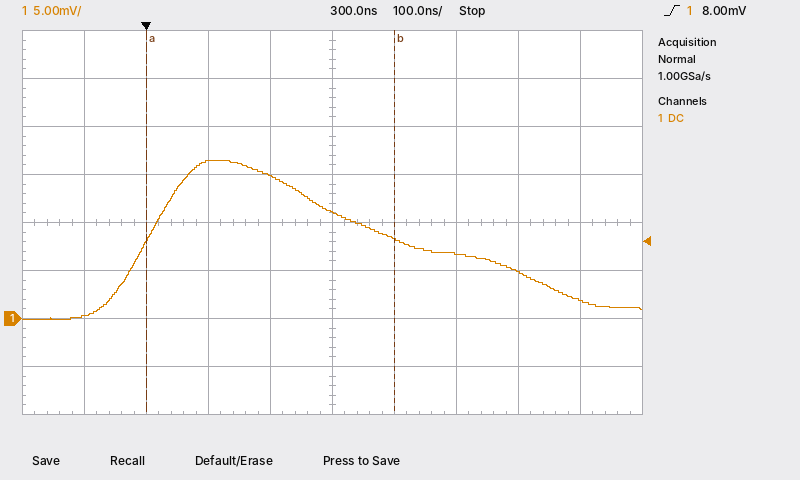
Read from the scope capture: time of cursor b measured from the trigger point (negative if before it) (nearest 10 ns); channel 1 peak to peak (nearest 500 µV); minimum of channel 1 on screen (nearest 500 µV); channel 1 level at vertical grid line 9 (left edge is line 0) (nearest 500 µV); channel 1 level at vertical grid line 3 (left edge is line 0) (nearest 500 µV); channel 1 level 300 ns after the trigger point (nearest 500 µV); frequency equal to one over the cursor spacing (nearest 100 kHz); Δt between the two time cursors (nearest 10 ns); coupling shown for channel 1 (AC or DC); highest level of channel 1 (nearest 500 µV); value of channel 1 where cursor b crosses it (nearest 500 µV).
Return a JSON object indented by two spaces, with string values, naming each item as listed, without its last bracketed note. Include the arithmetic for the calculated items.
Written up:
{
  "time of cursor b measured from the trigger point (negative if before it)": "+400 ns",
  "channel 1 peak to peak": "16.5 mV − (0.0 mV) = 16.5 mV",
  "minimum of channel 1 on screen": "0.0 mV",
  "channel 1 level at vertical grid line 9 (left edge is line 0)": "2.0 mV",
  "channel 1 level at vertical grid line 3 (left edge is line 0)": "16.5 mV",
  "channel 1 level 300 ns after the trigger point": "11.0 mV",
  "frequency equal to one over the cursor spacing": "1 / 400 ns ≈ 2.5 MHz",
  "Δt between the two time cursors": "400 ns",
  "coupling shown for channel 1": "DC",
  "highest level of channel 1": "16.5 mV",
  "value of channel 1 where cursor b crosses it": "8.5 mV"
}
